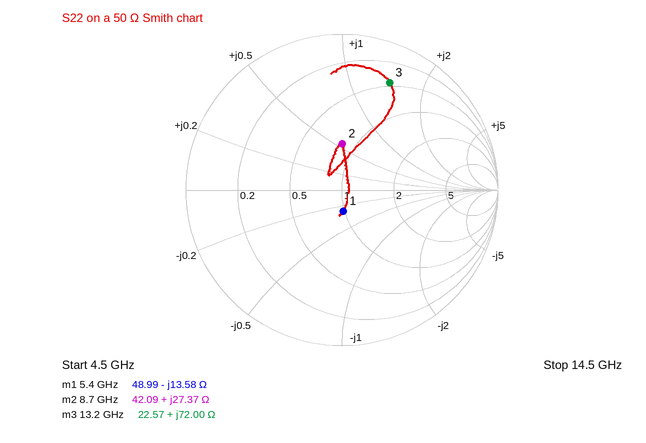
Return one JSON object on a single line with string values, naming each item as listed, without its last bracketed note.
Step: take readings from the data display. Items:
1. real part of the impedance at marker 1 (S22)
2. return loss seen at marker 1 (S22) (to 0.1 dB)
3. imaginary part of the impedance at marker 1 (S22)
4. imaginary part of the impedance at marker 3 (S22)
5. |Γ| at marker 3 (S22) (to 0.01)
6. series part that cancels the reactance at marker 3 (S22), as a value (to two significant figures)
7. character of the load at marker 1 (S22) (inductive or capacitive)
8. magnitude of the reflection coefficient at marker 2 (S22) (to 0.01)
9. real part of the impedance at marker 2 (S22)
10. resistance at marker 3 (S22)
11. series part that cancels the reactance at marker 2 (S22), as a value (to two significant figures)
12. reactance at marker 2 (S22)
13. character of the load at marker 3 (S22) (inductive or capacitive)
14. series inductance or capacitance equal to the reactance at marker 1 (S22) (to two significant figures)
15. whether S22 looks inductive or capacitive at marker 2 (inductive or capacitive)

{"real part of the impedance at marker 1": "48.99 Ω", "return loss seen at marker 1 (S22)": "17.3 dB", "imaginary part of the impedance at marker 1": "-13.58 Ω", "imaginary part of the impedance at marker 3": "+72.00 Ω", "|Γ| at marker 3 (S22)": "0.75", "series part that cancels the reactance at marker 3 (S22), as a value": "170 fF", "character of the load at marker 1 (S22)": "capacitive", "magnitude of the reflection coefficient at marker 2 (S22)": "0.30", "real part of the impedance at marker 2": "42.09 Ω", "resistance at marker 3": "22.57 Ω", "series part that cancels the reactance at marker 2 (S22), as a value": "670 fF", "reactance at marker 2": "+27.37 Ω", "character of the load at marker 3 (S22)": "inductive", "series inductance or capacitance equal to the reactance at marker 1 (S22)": "2.2 pF", "whether S22 looks inductive or capacitive at marker 2": "inductive"}
